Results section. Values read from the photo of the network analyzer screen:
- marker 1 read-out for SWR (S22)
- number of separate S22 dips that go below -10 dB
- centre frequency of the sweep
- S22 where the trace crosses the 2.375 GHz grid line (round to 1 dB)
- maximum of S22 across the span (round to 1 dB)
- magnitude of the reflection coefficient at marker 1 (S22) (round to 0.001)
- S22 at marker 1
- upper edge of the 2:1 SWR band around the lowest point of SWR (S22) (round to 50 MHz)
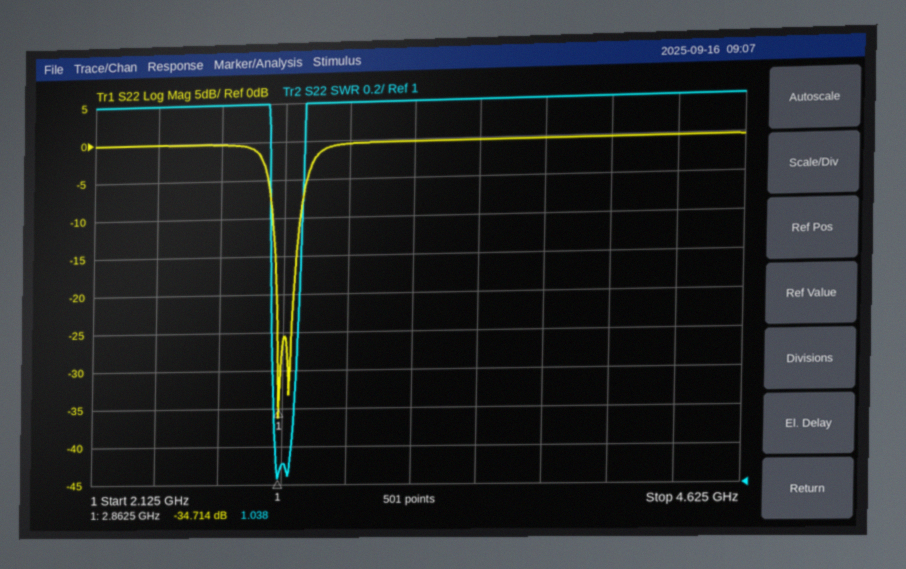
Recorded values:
1.038
2
3.375 GHz
0 dB
0 dB
0.018
-34.714 dB
2.95 GHz
